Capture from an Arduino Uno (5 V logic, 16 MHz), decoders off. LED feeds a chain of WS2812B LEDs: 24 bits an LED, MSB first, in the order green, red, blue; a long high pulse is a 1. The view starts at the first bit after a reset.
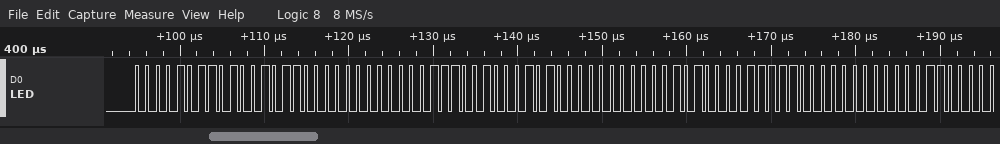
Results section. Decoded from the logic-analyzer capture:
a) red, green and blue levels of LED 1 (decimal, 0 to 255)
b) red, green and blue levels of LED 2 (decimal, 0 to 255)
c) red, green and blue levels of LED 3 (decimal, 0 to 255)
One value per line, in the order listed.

75, 11, 0
69, 14, 0
62, 20, 0
